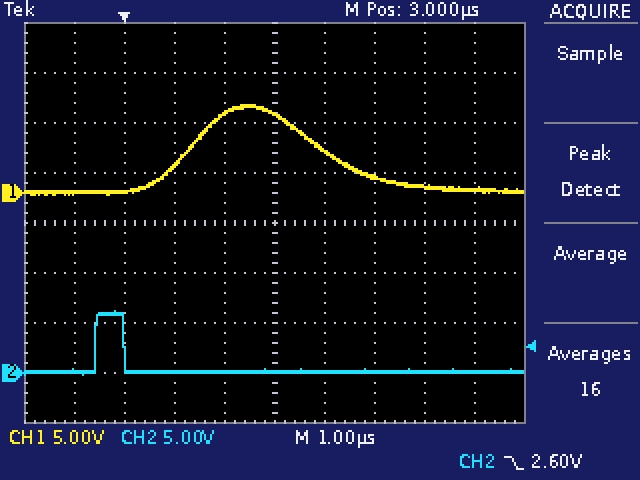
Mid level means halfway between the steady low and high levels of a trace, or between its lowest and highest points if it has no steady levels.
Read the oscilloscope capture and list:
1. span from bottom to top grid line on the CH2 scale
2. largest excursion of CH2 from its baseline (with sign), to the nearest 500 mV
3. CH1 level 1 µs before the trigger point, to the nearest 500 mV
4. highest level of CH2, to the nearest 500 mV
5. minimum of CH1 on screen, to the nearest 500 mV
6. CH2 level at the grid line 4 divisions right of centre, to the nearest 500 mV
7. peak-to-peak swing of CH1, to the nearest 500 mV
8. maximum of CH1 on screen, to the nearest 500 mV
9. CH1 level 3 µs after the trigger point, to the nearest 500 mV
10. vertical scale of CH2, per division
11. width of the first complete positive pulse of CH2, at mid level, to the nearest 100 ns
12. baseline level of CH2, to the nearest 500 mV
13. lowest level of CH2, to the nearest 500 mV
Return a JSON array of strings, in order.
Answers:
["40 V", "+6.0 V", "0.0 V", "6.0 V", "0.0 V", "0.0 V", "9.0 V", "9.0 V", "8.0 V", "5 V", "600 ns", "0.0 V", "0.0 V"]
